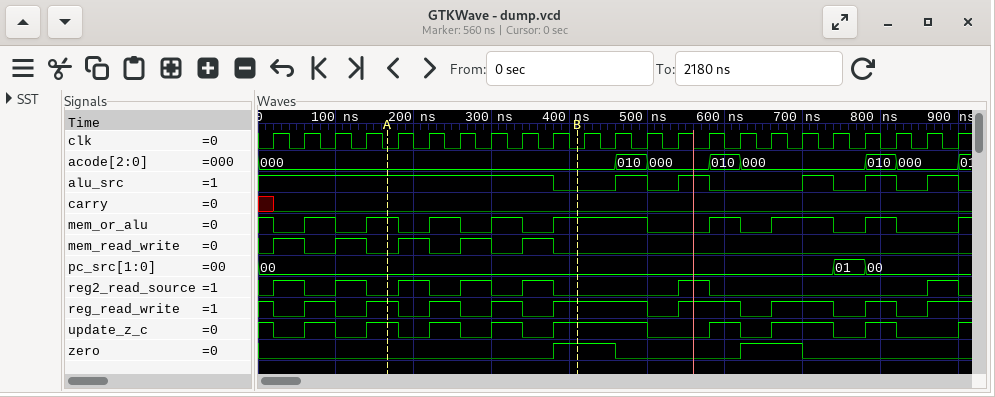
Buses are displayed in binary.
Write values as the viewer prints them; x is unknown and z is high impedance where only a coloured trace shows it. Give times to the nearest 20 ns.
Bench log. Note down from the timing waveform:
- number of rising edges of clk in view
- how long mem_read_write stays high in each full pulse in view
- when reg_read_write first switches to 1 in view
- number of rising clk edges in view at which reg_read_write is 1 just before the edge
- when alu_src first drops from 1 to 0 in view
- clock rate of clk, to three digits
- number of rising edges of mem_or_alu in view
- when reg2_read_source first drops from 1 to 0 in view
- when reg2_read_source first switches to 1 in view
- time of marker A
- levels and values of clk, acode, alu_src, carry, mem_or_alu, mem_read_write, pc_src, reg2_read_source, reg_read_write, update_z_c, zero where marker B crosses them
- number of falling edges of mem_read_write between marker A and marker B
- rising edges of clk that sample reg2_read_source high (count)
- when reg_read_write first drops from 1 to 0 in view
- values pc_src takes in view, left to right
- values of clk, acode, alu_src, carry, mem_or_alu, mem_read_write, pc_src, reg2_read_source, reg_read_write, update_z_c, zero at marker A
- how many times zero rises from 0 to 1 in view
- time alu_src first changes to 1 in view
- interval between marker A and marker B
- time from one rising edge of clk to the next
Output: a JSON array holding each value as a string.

["23", "40 ns, 40 ns, 40 ns, 40 ns, 40 ns", "60 ns", "14", "380 ns", "25.0 MHz", "9", "60 ns", "20 ns", "160 ns", "clk=0, acode=000, alu_src=0, carry=0, mem_or_alu=1, mem_read_write=0, pc_src=00, reg2_read_source=0, reg_read_write=1, update_z_c=1, zero=1", "3", "7", "20 ns", "00, 01, 00", "clk=0, acode=000, alu_src=1, carry=0, mem_or_alu=1, mem_read_write=0, pc_src=00, reg2_read_source=0, reg_read_write=1, update_z_c=1, zero=0", "2", "460 ns", "240 ns", "40 ns"]
